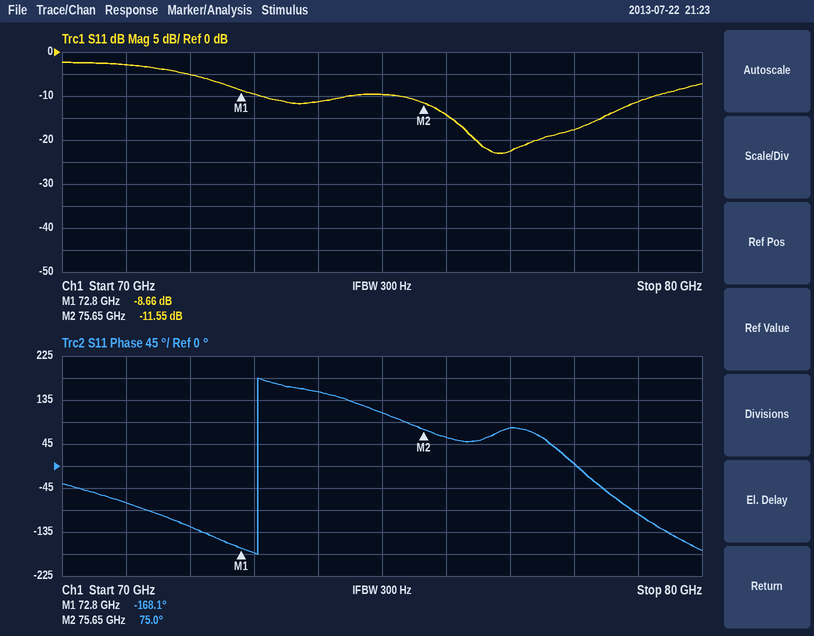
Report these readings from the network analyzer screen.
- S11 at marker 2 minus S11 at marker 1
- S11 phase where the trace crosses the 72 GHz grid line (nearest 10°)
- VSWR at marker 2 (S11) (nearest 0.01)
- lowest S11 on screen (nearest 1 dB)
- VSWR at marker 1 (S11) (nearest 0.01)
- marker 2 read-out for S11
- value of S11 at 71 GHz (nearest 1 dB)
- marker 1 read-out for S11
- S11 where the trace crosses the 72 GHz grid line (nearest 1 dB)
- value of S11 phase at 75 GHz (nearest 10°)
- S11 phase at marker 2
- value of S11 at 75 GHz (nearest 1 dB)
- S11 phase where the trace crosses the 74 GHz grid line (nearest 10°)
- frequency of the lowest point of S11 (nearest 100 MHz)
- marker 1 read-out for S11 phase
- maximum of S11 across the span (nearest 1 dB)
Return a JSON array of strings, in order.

["-2.89 dB", "-120°", "1.72", "-23 dB", "2.17", "-11.55 dB", "-3 dB", "-8.66 dB", "-5 dB", "110°", "75.0°", "-10 dB", "150°", "76.8 GHz", "-168.1°", "-2 dB"]
